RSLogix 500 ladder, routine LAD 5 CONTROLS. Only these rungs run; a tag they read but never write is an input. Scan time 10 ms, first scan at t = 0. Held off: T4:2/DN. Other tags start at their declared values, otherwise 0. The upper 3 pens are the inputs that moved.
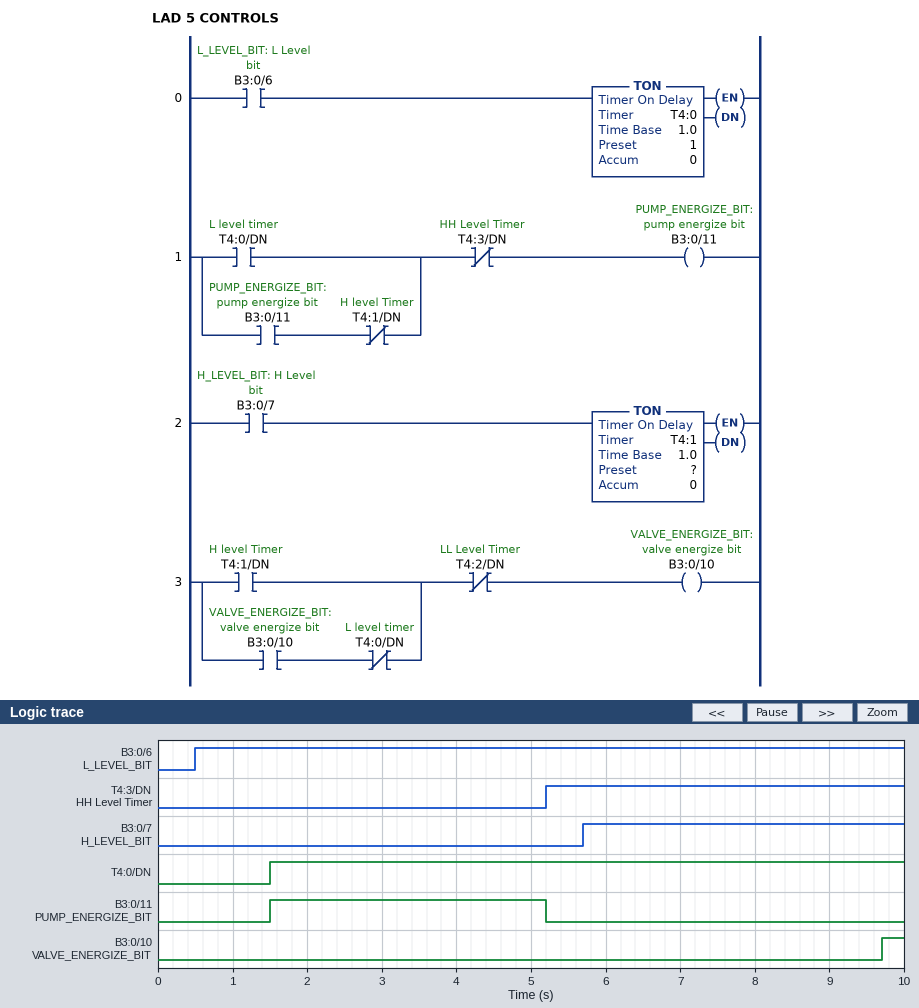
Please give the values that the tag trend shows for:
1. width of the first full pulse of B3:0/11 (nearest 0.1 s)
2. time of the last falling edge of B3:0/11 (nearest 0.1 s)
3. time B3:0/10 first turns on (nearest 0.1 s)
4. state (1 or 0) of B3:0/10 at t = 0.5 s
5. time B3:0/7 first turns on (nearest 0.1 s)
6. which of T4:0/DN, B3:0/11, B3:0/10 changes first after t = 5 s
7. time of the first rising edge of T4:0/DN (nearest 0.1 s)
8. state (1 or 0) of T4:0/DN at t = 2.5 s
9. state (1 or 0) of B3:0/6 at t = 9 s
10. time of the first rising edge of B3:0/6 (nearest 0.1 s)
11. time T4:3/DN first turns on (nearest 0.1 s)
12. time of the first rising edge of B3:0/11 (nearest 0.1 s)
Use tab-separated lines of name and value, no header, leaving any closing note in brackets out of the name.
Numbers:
width of the first full pulse of B3:0/11	3.7 s
time of the last falling edge of B3:0/11	5.2 s
time B3:0/10 first turns on	9.7 s
state (1 or 0) of B3:0/10 at t = 0.5 s	0
time B3:0/7 first turns on	5.7 s
which of T4:0/DN, B3:0/11, B3:0/10 changes first after t = 5 s	B3:0/11
time of the first rising edge of T4:0/DN	1.5 s
state (1 or 0) of T4:0/DN at t = 2.5 s	1
state (1 or 0) of B3:0/6 at t = 9 s	1
time of the first rising edge of B3:0/6	0.5 s
time T4:3/DN first turns on	5.2 s
time of the first rising edge of B3:0/11	1.5 s
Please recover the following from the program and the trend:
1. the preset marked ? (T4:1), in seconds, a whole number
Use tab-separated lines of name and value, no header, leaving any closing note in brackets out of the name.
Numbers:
the preset marked ? (T4:1), in seconds, a whole number	4 s
